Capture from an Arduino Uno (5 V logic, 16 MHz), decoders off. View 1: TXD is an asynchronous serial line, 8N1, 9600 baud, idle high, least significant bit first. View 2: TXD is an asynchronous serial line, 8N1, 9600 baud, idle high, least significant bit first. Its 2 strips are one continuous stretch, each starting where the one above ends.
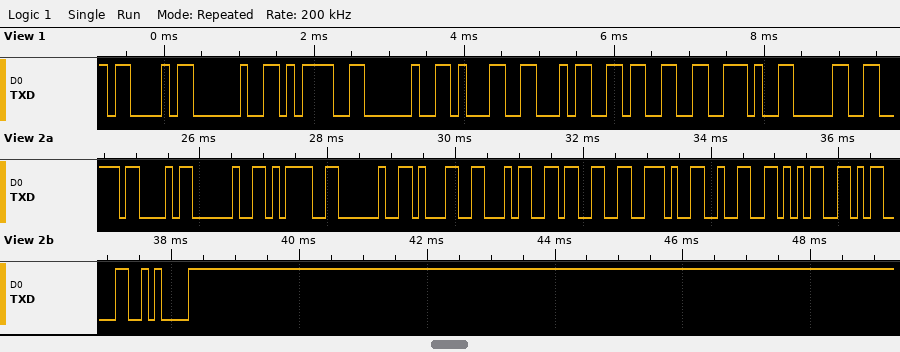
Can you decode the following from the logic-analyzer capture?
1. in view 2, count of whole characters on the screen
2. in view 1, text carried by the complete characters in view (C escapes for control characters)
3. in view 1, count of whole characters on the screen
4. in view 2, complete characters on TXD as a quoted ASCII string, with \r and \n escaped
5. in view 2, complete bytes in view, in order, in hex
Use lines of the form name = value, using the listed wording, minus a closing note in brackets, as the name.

in view 2, count of whole characters on the screen = 12
in view 1, text carried by the complete characters in view = "C = 143.0"
in view 1, count of whole characters on the screen = 9
in view 2, complete characters on TXD as a quoted ASCII string, with \r and \n escaped = "C = 143.25\r\n"
in view 2, complete bytes in view, in order, in hex = 43 20 3D 20 31 34 33 2E 32 35 0D 0A
